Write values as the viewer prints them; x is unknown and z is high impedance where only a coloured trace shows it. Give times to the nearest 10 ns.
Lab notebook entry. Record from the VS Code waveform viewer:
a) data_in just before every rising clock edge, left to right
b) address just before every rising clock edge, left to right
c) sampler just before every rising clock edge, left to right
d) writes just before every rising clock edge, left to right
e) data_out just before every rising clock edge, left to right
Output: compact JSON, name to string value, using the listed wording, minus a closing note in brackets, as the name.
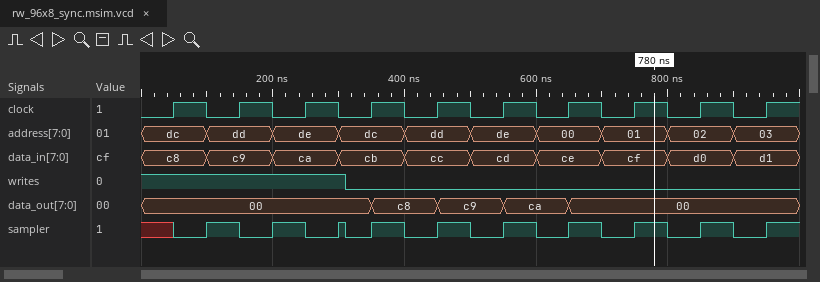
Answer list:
{"data_in just before every rising clock edge, left to right": "c8, c9, ca, cb, cc, cd, ce, cf, d0, d1", "address just before every rising clock edge, left to right": "dc, dd, de, dc, dd, de, 00, 01, 02, 03", "sampler just before every rising clock edge, left to right": "x 1 1 0 0 0 0 0 0 0", "writes just before every rising clock edge, left to right": "1 1 1 0 0 0 0 0 0 0", "data_out just before every rising clock edge, left to right": "00, 00, 00, 00, c8, c9, ca, 00, 00, 00"}
